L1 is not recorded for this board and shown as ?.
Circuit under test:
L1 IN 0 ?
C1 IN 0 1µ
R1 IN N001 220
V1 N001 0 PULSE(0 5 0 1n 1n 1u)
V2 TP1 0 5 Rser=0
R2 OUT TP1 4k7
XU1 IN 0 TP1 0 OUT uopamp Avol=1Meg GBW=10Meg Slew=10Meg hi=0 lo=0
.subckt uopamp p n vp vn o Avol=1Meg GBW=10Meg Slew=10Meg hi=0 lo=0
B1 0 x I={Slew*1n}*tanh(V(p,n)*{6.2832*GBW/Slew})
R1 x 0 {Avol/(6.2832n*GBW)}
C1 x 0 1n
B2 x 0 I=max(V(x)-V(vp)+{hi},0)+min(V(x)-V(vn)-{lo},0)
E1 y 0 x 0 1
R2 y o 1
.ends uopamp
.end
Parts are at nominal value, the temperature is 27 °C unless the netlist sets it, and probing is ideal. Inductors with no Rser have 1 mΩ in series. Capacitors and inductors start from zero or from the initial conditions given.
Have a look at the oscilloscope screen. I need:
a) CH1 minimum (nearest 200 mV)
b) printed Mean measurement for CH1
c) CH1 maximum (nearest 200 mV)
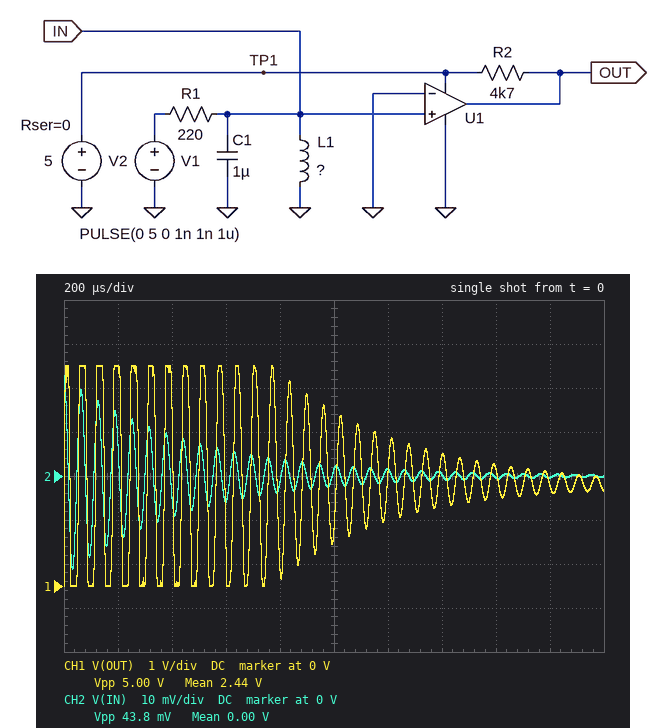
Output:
0 V
2.44 V
5.0 V
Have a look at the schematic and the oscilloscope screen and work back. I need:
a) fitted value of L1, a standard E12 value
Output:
100 µH
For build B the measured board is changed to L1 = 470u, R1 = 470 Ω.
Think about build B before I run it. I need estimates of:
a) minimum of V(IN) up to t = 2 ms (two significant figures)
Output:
-9.9 mV
